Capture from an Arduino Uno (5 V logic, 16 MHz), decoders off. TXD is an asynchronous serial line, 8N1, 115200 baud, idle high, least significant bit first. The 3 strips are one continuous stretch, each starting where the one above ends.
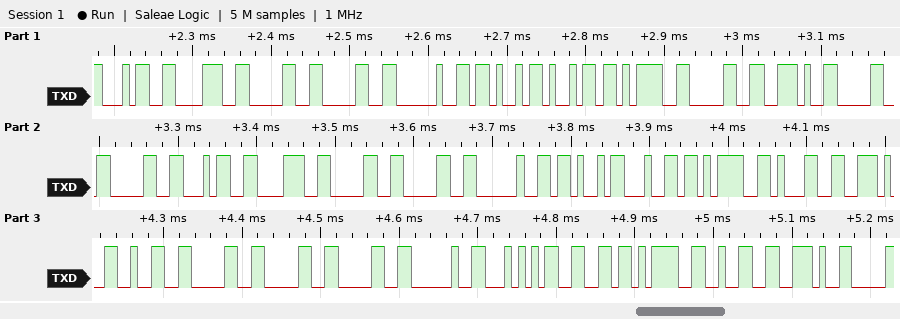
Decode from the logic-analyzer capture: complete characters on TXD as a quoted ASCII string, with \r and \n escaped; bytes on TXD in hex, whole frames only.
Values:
"4800 Ki=0.004800 Kd=1.2000 Tf=2."
34 38 30 30 20 4B 69 3D 30 2E 30 30 34 38 30 30 20 4B 64 3D 31 2E 32 30 30 30 20 54 66 3D 32 2E
